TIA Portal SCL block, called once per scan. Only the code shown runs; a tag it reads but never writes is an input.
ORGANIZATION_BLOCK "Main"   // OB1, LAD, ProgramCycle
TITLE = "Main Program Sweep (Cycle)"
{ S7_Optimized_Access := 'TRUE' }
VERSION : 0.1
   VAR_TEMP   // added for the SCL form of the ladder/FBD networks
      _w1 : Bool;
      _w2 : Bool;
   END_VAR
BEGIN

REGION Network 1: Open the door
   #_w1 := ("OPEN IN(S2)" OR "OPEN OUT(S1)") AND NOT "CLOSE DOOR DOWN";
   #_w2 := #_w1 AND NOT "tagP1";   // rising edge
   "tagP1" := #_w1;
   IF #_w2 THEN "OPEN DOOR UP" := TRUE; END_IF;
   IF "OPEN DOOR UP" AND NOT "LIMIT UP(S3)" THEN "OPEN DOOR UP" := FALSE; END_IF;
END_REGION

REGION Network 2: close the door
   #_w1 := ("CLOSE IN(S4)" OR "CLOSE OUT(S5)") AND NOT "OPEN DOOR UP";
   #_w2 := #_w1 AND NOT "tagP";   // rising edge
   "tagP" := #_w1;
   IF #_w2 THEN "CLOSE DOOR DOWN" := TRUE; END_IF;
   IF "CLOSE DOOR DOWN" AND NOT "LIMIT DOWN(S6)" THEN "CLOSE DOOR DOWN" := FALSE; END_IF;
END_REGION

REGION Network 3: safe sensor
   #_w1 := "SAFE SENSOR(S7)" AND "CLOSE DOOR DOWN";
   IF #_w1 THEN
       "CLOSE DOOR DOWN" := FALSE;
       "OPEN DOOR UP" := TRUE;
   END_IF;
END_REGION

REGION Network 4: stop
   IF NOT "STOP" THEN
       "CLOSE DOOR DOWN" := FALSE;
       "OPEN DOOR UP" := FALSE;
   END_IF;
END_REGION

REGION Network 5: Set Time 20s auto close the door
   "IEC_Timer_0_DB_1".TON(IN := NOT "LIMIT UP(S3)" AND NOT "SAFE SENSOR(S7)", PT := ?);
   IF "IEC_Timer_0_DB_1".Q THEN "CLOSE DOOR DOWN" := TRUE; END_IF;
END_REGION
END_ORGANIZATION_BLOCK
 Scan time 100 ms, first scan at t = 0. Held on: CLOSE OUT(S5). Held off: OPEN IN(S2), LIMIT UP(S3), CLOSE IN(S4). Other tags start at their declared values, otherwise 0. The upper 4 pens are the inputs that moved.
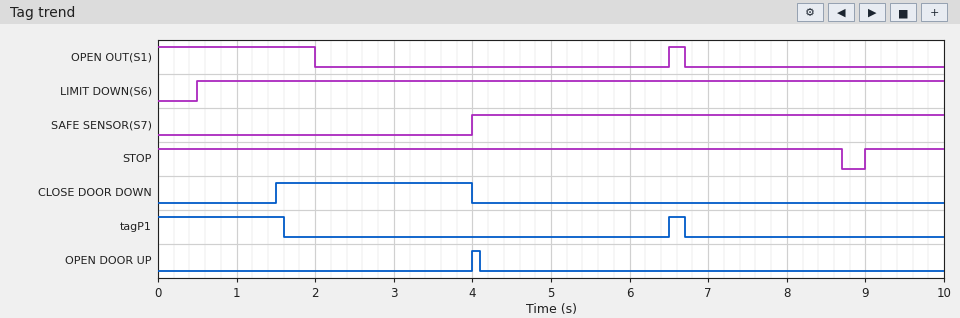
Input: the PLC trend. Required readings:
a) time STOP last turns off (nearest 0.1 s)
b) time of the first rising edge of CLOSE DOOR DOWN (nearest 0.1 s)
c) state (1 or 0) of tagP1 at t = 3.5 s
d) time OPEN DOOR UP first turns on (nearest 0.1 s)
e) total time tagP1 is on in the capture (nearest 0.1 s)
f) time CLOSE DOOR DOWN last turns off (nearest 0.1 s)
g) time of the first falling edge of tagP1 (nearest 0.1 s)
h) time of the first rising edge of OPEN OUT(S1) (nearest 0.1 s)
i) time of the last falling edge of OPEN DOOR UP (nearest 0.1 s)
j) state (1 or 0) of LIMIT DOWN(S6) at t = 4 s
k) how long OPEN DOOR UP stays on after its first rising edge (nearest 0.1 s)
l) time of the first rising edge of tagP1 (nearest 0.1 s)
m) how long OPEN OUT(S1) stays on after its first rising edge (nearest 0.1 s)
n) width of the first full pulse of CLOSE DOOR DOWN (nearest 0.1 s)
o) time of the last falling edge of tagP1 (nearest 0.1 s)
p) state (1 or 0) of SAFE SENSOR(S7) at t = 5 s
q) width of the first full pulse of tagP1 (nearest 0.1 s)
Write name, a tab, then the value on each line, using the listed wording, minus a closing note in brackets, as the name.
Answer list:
time STOP last turns off	8.7 s
time of the first rising edge of CLOSE DOOR DOWN	1.5 s
state (1 or 0) of tagP1 at t = 3.5 s	0
time OPEN DOOR UP first turns on	4.0 s
total time tagP1 is on in the capture	1.8 s
time CLOSE DOOR DOWN last turns off	4.0 s
time of the first falling edge of tagP1	1.6 s
time of the first rising edge of OPEN OUT(S1)	6.5 s
time of the last falling edge of OPEN DOOR UP	4.1 s
state (1 or 0) of LIMIT DOWN(S6) at t = 4 s	1
how long OPEN DOOR UP stays on after its first rising edge	0.1 s
time of the first rising edge of tagP1	6.5 s
how long OPEN OUT(S1) stays on after its first rising edge	0.2 s
width of the first full pulse of CLOSE DOOR DOWN	2.5 s
time of the last falling edge of tagP1	6.7 s
state (1 or 0) of SAFE SENSOR(S7) at t = 5 s	1
width of the first full pulse of tagP1	0.2 s
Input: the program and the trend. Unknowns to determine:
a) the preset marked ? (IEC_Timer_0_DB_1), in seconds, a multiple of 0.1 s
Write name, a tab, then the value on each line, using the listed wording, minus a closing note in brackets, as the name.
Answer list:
the preset marked ? (IEC_Timer_0_DB_1), in seconds, a multiple of 0.1 s	1.5 s
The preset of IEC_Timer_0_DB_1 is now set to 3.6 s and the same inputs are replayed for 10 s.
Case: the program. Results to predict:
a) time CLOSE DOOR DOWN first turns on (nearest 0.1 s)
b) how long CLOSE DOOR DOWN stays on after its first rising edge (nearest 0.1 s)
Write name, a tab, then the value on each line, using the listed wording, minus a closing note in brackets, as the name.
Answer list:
time CLOSE DOOR DOWN first turns on	3.6 s
how long CLOSE DOOR DOWN stays on after its first rising edge	0.4 s
